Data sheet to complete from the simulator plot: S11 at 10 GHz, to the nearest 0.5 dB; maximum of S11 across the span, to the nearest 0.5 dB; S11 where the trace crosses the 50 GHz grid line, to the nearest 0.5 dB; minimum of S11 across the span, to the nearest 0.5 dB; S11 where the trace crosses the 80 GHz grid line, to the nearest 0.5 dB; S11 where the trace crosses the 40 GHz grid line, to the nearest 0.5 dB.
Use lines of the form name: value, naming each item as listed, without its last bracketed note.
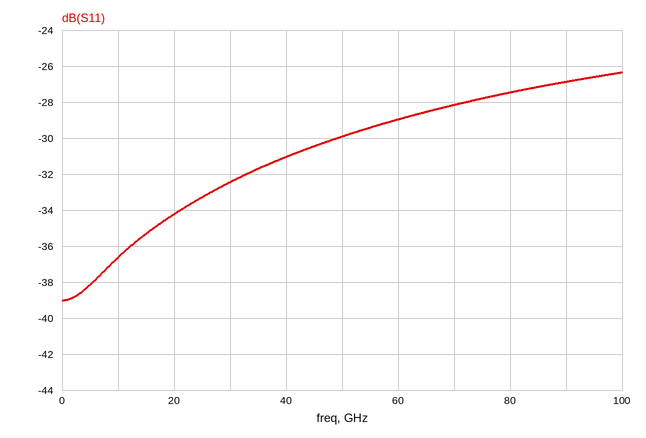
S11 at 10 GHz, to the nearest 0.5 dB: -36.5 dB
maximum of S11 across the span, to the nearest 0.5 dB: -26.5 dB
S11 where the trace crosses the 50 GHz grid line, to the nearest 0.5 dB: -30.0 dB
minimum of S11 across the span, to the nearest 0.5 dB: -39.0 dB
S11 where the trace crosses the 80 GHz grid line, to the nearest 0.5 dB: -27.5 dB
S11 where the trace crosses the 40 GHz grid line, to the nearest 0.5 dB: -31.0 dB
